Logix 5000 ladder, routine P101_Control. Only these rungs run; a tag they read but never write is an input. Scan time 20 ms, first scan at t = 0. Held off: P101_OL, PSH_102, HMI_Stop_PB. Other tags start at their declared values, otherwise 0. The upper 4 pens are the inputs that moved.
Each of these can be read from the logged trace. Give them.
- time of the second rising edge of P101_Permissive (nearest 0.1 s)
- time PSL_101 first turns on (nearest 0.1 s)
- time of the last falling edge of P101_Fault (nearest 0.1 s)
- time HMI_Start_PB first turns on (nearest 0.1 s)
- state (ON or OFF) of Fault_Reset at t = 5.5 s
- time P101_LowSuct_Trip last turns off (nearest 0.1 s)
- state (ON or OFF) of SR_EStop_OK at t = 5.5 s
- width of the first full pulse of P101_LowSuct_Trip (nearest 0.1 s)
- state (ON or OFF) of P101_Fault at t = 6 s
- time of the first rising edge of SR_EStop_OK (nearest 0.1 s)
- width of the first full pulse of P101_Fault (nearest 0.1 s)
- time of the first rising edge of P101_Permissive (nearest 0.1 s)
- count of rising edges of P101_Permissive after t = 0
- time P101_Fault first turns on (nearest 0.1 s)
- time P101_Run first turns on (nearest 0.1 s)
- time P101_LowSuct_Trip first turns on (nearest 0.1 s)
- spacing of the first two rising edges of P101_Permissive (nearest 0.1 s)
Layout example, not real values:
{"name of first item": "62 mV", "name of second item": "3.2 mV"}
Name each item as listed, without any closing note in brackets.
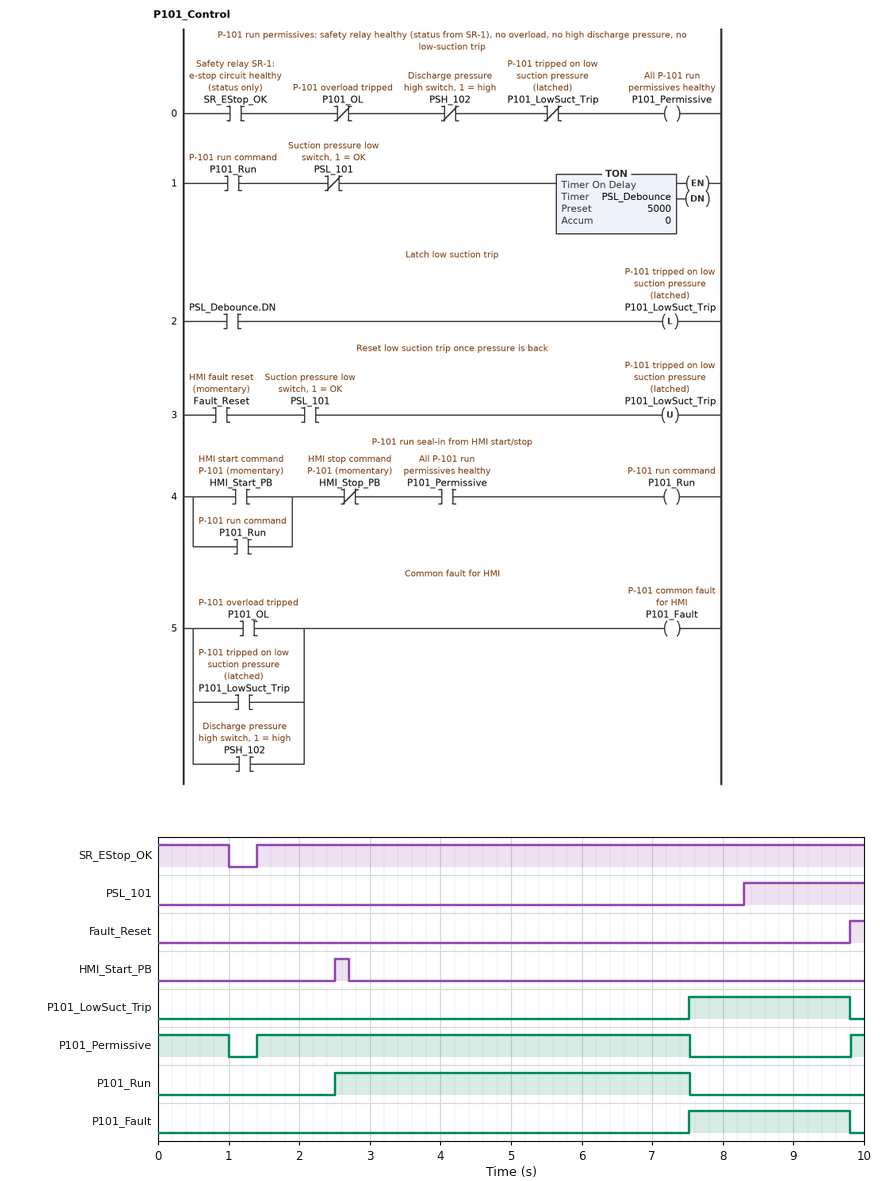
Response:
{"time of the second rising edge of P101_Permissive": "9.8 s", "time PSL_101 first turns on": "8.3 s", "time of the last falling edge of P101_Fault": "9.8 s", "time HMI_Start_PB first turns on": "2.5 s", "state (ON or OFF) of Fault_Reset at t = 5.5 s": "OFF", "time P101_LowSuct_Trip last turns off": "9.8 s", "state (ON or OFF) of SR_EStop_OK at t = 5.5 s": "ON", "width of the first full pulse of P101_LowSuct_Trip": "2.3 s", "state (ON or OFF) of P101_Fault at t = 6 s": "OFF", "time of the first rising edge of SR_EStop_OK": "1.4 s", "width of the first full pulse of P101_Fault": "2.3 s", "time of the first rising edge of P101_Permissive": "1.4 s", "count of rising edges of P101_Permissive after t = 0": "2", "time P101_Fault first turns on": "7.5 s", "time P101_Run first turns on": "2.5 s", "time P101_LowSuct_Trip first turns on": "7.5 s", "spacing of the first two rising edges of P101_Permissive": "8.4 s"}
